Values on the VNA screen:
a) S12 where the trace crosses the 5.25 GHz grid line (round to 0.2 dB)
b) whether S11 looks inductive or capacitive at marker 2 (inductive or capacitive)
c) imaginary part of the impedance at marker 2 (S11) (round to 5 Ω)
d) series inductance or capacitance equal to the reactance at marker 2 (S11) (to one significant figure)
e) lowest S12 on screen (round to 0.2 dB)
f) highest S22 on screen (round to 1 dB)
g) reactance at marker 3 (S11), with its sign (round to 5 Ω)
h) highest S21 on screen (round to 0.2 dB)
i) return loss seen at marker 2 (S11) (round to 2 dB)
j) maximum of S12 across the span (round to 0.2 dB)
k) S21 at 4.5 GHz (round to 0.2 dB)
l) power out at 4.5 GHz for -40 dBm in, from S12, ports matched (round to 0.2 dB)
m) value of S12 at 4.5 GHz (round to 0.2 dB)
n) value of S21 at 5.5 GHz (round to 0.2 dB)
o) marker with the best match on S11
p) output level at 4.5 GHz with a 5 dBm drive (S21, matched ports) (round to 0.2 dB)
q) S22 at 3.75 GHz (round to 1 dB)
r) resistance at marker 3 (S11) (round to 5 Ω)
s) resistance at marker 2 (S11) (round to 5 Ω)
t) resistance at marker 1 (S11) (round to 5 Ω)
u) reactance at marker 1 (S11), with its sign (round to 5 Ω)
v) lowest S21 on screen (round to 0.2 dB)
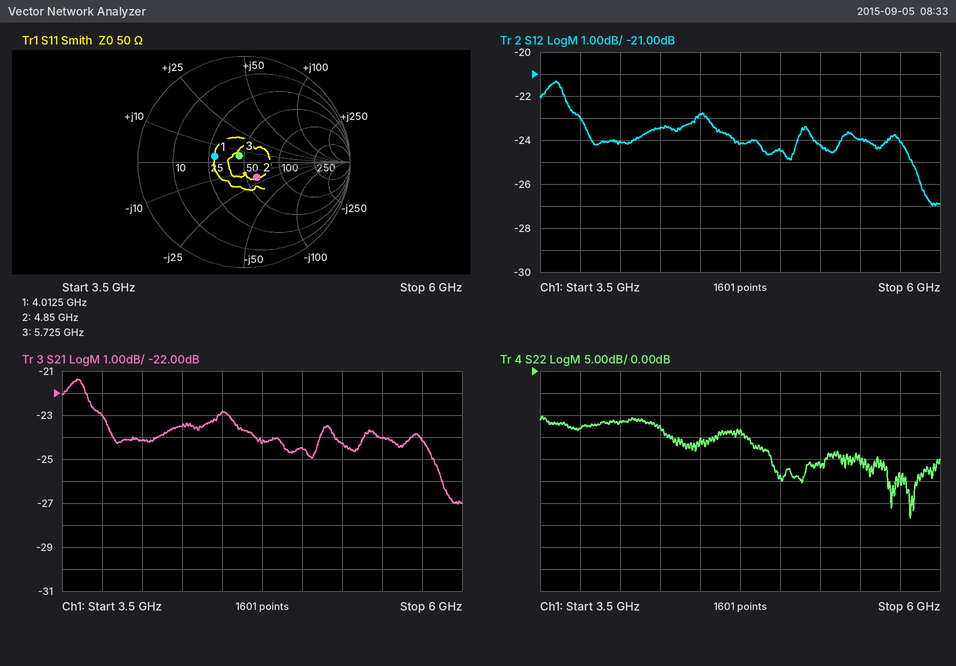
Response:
-24.2 dB
capacitive
-20 Ω
2 pF
-27.0 dB
-10 dB
+5 Ω
-21.4 dB
14 dB
-21.4 dB
-22.8 dB
-62.8 dBm
-22.8 dB
-24.0 dB
marker 3
-17.8 dBm
-13 dB
45 Ω
60 Ω
30 Ω
+5 Ω
-27.0 dB
